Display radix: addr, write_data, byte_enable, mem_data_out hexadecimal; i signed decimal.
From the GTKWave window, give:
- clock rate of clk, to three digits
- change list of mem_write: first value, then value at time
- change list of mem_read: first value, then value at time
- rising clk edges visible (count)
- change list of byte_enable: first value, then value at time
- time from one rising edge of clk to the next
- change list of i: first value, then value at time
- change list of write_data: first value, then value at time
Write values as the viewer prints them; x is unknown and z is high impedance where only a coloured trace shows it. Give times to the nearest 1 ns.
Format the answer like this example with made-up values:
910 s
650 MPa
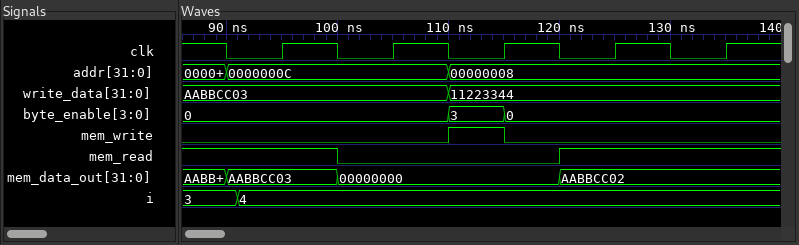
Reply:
100 MHz
0, 1 at 110 ns, 0 at 115 ns
1, 0 at 100 ns, 1 at 120 ns
5
0, 3 at 110 ns, 0 at 115 ns
10 ns
3, 4 at 91 ns
AABBCC03, 11223344 at 110 ns
